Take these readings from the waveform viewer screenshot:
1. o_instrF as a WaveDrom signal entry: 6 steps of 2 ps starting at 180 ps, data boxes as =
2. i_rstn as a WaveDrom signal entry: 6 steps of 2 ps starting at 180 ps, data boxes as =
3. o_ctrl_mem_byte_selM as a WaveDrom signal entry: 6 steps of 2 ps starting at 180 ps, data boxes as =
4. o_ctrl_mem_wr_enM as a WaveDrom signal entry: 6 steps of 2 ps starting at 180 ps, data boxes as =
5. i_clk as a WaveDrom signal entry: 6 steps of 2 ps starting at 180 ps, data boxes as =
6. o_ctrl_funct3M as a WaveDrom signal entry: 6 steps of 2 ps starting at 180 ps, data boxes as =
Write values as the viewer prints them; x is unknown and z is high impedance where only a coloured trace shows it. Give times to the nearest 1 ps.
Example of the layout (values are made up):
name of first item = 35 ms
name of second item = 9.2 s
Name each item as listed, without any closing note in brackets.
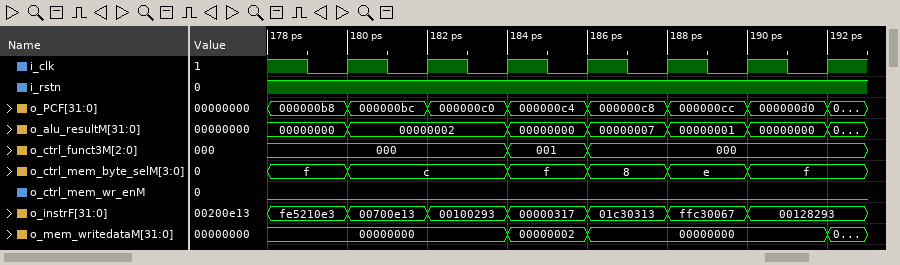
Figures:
o_instrF as a WaveDrom signal entry: 6 steps of 2 ps starting at 180 ps, data boxes as = = {name: 'o_instrF', wave: '======', data: '00700e13 00100293 00000317 01c30313 ffc30067 00128293'}
i_rstn as a WaveDrom signal entry: 6 steps of 2 ps starting at 180 ps, data boxes as = = {name: 'i_rstn', wave: '1.....'}
o_ctrl_mem_byte_selM as a WaveDrom signal entry: 6 steps of 2 ps starting at 180 ps, data boxes as = = {name: 'o_ctrl_mem_byte_selM', wave: '=.====', data: 'c f 8 e f'}
o_ctrl_mem_wr_enM as a WaveDrom signal entry: 6 steps of 2 ps starting at 180 ps, data boxes as = = {name: 'o_ctrl_mem_wr_enM', wave: '0.....'}
i_clk as a WaveDrom signal entry: 6 steps of 2 ps starting at 180 ps, data boxes as = = {name: 'i_clk', wave: 'p.....'}
o_ctrl_funct3M as a WaveDrom signal entry: 6 steps of 2 ps starting at 180 ps, data boxes as = = {name: 'o_ctrl_funct3M', wave: '=.==..', data: '000 001 000'}
